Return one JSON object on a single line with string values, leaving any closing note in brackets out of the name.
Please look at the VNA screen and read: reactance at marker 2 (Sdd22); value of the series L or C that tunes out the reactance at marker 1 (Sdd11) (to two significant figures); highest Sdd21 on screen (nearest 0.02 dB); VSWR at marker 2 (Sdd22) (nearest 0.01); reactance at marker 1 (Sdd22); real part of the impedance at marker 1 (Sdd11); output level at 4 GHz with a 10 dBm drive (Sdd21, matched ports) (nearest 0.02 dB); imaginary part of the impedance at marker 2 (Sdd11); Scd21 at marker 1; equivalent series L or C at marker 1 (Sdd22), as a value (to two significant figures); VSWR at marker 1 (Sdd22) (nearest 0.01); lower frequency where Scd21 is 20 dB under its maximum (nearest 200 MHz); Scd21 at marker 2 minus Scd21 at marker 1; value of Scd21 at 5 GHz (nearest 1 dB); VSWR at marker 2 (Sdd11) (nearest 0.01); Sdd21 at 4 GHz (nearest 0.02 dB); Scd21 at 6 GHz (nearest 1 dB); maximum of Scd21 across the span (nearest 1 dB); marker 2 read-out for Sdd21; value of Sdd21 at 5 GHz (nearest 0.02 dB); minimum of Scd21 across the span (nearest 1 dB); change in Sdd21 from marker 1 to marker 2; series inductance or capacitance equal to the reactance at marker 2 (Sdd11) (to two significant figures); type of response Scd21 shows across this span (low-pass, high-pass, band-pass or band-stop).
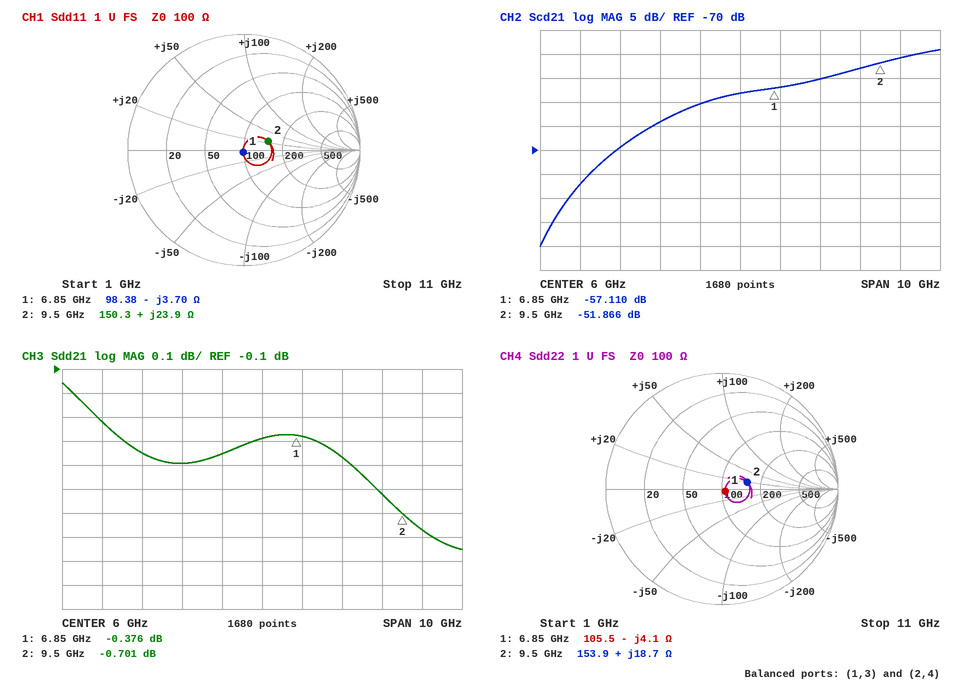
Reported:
{"reactance at marker 2": "+18.7 Ω", "value of the series L or C that tunes out the reactance at marker 1 (Sdd11)": "86 pH", "highest Sdd21 on screen": "-0.16 dB", "VSWR at marker 2 (Sdd22)": "1.58", "reactance at marker 1": "-4.1 Ω", "real part of the impedance at marker 1": "98.38 Ω", "output level at 4 GHz with a 10 dBm drive (Sdd21, matched ports)": "9.50 dBm", "imaginary part of the impedance at marker 2": "+23.9 Ω", "Scd21 at marker 1": "-57.110 dB", "equivalent series L or C at marker 1 (Sdd22), as a value": "5.7 pF", "VSWR at marker 1 (Sdd22)": "1.07", "lower frequency where Scd21 is 20 dB under its maximum": "3.0 GHz", "Scd21 at marker 2 minus Scd21 at marker 1": "5.244 dB", "value of Scd21 at 5 GHz": "-60 dB", "VSWR at marker 2 (Sdd11)": "1.57", "Sdd21 at 4 GHz": "-0.50 dB", "Scd21 at 6 GHz": "-58 dB", "maximum of Scd21 across the span": "-49 dB", "marker 2 read-out for Sdd21": "-0.701 dB", "value of Sdd21 at 5 GHz": "-0.46 dB", "minimum of Scd21 across the span": "-90 dB", "change in Sdd21 from marker 1 to marker 2": "-0.325 dB", "series inductance or capacitance equal to the reactance at marker 2 (Sdd11)": "400 pH", "type of response Scd21 shows across this span": "high-pass"}
